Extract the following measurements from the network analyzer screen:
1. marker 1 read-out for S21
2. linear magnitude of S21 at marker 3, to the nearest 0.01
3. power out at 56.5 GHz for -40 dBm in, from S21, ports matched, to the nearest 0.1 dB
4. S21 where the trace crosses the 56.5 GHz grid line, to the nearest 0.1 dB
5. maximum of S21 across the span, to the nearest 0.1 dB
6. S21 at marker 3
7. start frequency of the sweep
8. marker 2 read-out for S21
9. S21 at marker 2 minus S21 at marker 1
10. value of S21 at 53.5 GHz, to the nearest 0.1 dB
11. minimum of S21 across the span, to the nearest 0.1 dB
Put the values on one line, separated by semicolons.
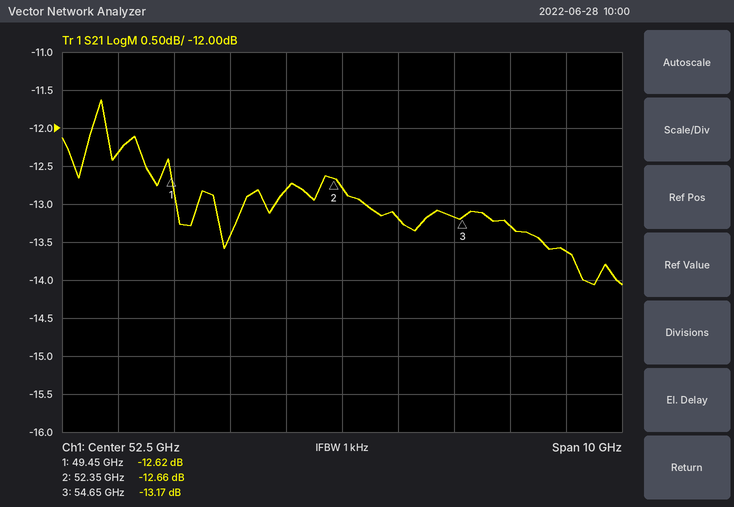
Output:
-12.62 dB; 0.22; -53.6 dBm; -13.6 dB; -11.6 dB; -13.17 dB; 47.5 GHz; -12.66 dB; -0.04 dB; -13.2 dB; -14.1 dB
